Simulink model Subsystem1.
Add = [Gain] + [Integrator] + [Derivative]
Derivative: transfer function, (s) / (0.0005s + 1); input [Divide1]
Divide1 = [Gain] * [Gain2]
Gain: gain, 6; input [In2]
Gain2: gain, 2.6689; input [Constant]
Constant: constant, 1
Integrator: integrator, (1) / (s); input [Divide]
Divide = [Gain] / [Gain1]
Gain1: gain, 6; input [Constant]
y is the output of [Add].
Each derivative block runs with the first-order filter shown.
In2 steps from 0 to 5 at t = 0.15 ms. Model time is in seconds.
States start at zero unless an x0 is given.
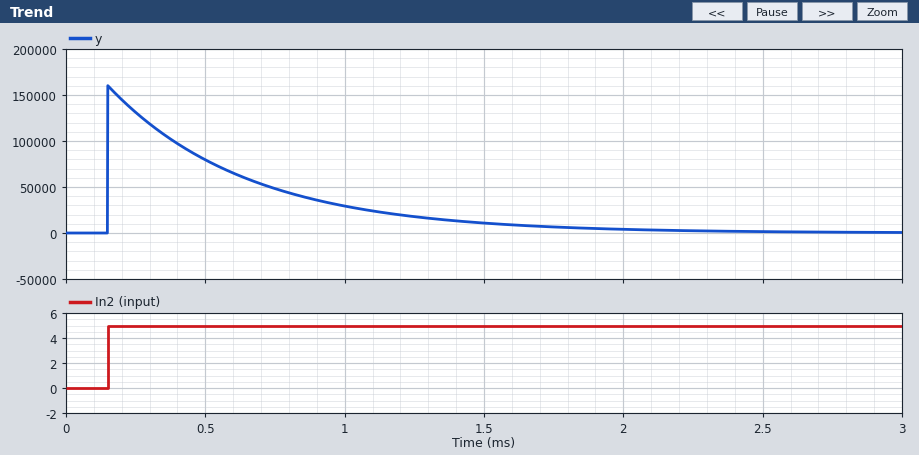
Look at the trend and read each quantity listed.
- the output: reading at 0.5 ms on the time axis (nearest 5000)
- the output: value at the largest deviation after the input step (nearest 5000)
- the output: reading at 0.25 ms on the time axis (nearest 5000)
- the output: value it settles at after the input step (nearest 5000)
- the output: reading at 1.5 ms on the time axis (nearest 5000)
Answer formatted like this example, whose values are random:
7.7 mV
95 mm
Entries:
80000
160000
130000
0
10000
